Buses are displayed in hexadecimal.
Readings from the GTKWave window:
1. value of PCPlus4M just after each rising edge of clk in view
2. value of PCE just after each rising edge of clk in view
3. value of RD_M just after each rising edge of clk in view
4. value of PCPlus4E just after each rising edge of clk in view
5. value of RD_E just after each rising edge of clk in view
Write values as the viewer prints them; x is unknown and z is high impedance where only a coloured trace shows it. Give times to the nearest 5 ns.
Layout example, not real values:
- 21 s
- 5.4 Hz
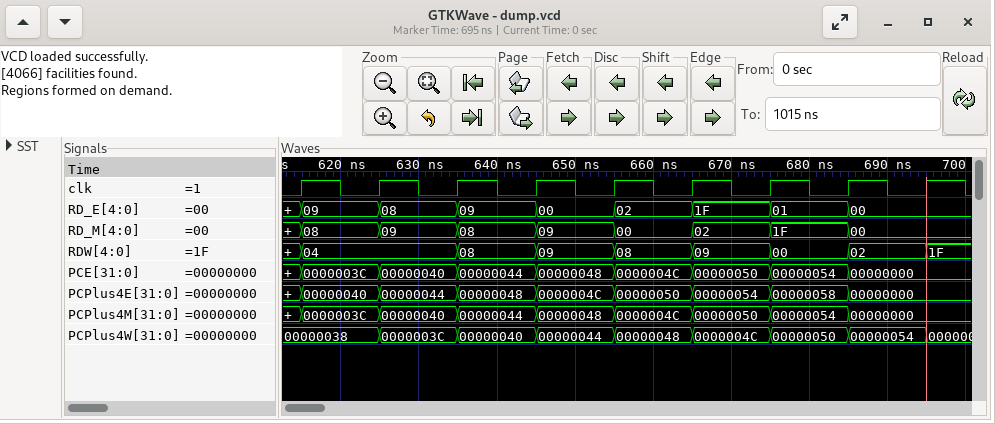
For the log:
- 0000003C, 00000040, 00000044, 00000048, 0000004C, 00000050, 00000054, 00000000, 00000000
- 0000003C, 00000040, 00000044, 00000048, 0000004C, 00000050, 00000054, 00000000, 00000000
- 08, 09, 08, 09, 00, 02, 1F, 00, 00
- 00000040, 00000044, 00000048, 0000004C, 00000050, 00000054, 00000058, 00000000, 00000000
- 09, 08, 09, 00, 02, 1F, 01, 00, 00
